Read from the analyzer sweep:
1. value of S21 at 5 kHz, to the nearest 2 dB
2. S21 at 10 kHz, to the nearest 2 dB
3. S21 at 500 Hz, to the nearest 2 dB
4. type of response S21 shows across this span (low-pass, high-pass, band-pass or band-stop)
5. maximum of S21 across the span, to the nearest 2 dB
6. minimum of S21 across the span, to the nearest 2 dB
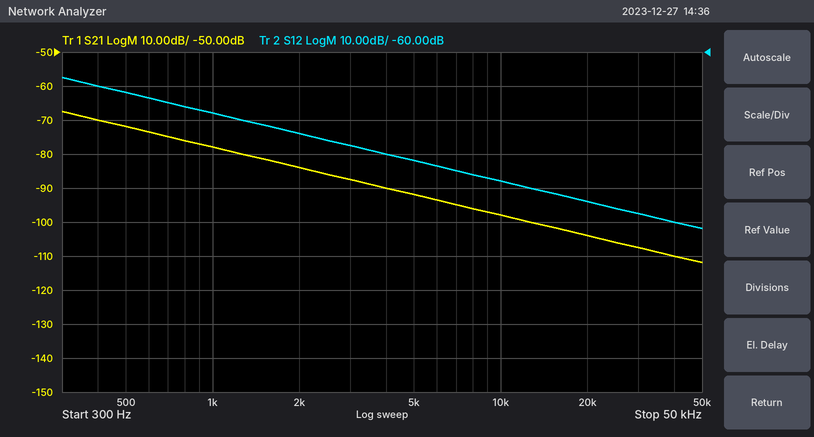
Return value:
-92 dB
-98 dB
-72 dB
low-pass
-68 dB
-112 dB
